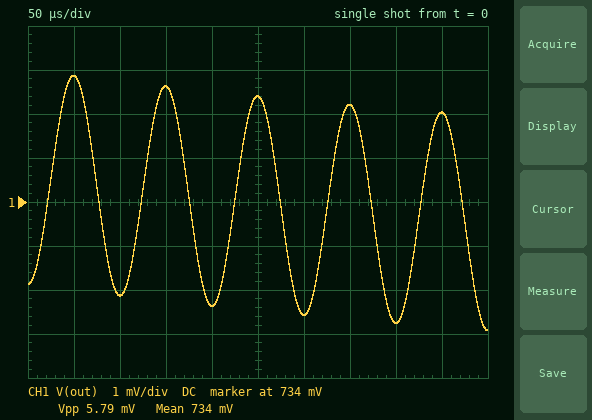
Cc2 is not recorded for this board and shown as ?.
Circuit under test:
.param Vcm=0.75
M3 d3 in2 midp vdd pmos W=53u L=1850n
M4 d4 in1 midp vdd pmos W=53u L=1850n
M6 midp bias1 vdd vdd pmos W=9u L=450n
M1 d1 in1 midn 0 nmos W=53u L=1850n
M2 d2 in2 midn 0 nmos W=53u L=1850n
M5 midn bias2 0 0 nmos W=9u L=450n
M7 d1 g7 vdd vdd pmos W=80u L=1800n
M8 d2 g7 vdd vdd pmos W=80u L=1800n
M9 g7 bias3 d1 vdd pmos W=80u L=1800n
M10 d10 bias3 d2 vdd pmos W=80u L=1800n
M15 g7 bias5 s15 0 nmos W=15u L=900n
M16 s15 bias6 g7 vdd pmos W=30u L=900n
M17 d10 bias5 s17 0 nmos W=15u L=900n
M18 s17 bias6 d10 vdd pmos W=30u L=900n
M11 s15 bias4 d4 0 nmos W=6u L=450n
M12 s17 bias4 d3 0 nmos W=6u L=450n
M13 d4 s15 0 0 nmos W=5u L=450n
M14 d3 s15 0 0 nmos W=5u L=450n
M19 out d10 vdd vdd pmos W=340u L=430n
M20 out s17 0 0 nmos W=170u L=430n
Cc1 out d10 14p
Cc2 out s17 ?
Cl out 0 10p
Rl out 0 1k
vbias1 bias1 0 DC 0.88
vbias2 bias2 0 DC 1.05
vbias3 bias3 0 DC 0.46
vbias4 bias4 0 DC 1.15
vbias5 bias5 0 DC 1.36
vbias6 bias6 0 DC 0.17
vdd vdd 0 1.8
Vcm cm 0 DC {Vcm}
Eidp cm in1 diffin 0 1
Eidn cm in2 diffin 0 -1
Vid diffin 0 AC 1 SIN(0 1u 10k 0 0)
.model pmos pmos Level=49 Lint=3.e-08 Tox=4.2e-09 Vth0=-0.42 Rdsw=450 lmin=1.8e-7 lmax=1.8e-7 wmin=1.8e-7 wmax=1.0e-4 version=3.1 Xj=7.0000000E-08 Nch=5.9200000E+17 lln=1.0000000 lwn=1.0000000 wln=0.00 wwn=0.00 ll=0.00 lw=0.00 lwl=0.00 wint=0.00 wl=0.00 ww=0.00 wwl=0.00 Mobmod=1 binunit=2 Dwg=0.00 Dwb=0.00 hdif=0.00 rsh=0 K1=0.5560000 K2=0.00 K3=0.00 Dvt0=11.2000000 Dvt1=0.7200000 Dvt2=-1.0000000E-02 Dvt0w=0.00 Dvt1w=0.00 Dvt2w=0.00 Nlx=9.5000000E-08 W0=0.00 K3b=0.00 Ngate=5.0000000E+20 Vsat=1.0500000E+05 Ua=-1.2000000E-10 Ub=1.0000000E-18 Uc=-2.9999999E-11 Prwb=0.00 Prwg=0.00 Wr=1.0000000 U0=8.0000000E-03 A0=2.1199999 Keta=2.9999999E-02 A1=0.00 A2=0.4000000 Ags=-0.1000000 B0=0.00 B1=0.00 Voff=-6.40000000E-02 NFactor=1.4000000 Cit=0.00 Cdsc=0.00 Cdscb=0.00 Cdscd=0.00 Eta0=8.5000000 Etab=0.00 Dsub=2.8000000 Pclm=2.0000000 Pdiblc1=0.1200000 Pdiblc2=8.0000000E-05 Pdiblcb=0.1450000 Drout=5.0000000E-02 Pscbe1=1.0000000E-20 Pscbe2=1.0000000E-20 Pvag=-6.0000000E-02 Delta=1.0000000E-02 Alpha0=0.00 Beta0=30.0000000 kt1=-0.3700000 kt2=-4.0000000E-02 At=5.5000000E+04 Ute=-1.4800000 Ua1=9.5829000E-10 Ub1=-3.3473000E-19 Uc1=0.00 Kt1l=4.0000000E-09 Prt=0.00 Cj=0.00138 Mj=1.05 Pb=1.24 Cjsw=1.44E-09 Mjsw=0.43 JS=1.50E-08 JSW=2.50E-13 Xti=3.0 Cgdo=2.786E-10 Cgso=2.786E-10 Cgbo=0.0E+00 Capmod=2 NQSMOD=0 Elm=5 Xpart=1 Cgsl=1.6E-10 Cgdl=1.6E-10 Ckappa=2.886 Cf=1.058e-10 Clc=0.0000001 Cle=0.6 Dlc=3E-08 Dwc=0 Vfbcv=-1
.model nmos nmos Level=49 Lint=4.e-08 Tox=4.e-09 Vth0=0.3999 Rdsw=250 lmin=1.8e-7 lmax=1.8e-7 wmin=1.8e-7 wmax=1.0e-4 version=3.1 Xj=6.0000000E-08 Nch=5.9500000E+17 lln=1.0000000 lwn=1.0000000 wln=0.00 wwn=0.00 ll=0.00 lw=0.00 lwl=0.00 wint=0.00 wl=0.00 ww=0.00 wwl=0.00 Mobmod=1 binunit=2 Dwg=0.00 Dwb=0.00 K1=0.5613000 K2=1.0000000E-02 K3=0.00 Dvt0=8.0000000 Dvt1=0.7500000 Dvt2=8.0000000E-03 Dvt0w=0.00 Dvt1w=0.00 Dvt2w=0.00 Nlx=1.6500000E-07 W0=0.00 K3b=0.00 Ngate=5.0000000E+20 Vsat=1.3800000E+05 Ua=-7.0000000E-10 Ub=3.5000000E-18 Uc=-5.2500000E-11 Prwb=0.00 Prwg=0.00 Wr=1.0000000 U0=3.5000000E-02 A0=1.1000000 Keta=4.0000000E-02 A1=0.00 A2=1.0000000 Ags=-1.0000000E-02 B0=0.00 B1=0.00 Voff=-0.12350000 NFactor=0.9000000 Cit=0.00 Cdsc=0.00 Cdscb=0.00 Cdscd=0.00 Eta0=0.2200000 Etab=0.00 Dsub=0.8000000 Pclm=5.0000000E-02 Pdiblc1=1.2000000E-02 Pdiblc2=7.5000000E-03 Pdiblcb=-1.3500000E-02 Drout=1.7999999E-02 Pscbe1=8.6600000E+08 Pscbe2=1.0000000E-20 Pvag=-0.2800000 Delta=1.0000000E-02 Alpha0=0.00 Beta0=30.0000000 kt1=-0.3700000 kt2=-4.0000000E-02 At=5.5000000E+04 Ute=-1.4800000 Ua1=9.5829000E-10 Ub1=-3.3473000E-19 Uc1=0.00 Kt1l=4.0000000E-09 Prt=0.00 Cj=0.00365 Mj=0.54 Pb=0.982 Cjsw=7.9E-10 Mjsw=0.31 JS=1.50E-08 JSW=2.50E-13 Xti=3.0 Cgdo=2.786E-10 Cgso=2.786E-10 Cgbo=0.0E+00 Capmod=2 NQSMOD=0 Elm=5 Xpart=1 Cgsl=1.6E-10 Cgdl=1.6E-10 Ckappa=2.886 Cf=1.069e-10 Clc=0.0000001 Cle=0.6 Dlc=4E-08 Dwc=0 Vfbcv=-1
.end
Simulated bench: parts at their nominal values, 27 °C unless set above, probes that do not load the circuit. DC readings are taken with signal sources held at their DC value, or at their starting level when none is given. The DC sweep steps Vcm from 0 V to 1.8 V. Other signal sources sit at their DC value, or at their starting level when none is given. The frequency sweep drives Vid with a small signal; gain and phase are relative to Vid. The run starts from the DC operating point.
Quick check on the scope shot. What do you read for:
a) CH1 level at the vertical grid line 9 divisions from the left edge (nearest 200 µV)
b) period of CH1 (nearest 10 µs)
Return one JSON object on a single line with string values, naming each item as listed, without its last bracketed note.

{"CH1 level at the vertical grid line 9 divisions from the left edge": "736.0 mV", "period of CH1": "100 µs"}
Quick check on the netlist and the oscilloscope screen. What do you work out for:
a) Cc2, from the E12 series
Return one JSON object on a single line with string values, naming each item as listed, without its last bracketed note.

{"Cc2, from the E12 series": "4.7 pF"}
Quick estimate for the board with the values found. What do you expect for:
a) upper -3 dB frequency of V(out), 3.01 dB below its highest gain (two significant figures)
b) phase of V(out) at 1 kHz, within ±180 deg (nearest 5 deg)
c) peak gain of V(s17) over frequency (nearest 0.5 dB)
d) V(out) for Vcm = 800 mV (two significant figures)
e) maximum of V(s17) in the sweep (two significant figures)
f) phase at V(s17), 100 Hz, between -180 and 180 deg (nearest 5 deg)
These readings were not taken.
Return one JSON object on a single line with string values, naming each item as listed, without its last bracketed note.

{"upper -3 dB frequency of V(out), 3.01 dB below its highest gain": "180 Hz", "phase of V(out) at 1 kHz, within ±180 deg": "-80 deg", "peak gain of V(s17) over frequency": "79.5 dB", "V(out) for Vcm = 800 mV": "1.0 V", "maximum of V(s17) in the sweep": "800 mV", "phase at V(s17), 100 Hz, between -180 and 180 deg": "150 deg"}
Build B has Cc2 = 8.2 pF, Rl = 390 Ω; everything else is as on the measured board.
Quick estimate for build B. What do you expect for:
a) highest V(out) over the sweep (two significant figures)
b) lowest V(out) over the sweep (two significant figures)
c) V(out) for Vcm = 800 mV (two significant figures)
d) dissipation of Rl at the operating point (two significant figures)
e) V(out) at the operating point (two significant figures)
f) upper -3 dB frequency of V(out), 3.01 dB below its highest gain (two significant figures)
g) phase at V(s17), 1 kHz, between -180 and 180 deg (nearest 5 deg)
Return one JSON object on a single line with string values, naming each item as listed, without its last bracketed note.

{"highest V(out) over the sweep": "1.5 V", "lowest V(out) over the sweep": "49 mV", "V(out) for Vcm = 800 mV": "600 mV", "dissipation of Rl at the operating point": "470 µW", "V(out) at the operating point": "430 mV", "upper -3 dB frequency of V(out), 3.01 dB below its highest gain": "250 Hz", "phase at V(s17), 1 kHz, between -180 and 180 deg": "105 deg"}
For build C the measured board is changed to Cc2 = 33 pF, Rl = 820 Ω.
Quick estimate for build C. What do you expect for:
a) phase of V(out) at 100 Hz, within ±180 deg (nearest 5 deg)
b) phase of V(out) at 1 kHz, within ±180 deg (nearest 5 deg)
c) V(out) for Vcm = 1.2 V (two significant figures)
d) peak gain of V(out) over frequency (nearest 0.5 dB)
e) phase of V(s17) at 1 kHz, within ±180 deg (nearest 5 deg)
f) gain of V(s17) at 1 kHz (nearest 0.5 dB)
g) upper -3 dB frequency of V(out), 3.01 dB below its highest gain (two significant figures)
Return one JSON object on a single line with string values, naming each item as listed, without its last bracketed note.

{"phase of V(out) at 100 Hz, within ±180 deg": "-50 deg", "phase of V(out) at 1 kHz, within ±180 deg": "-85 deg", "V(out) for Vcm = 1.2 V": "1.6 V", "peak gain of V(out) over frequency": "102.0 dB", "phase of V(s17) at 1 kHz, within ±180 deg": "95 deg", "gain of V(s17) at 1 kHz": "57.5 dB", "upper -3 dB frequency of V(out), 3.01 dB below its highest gain": "79 Hz"}
